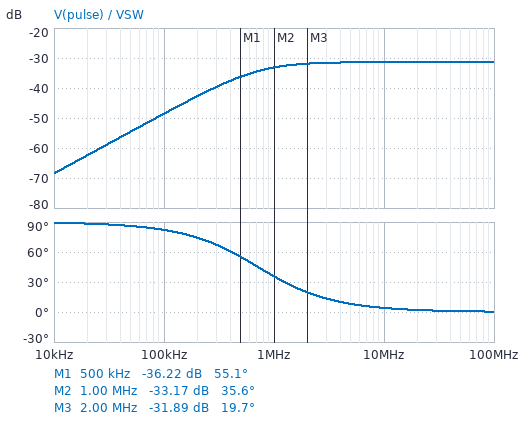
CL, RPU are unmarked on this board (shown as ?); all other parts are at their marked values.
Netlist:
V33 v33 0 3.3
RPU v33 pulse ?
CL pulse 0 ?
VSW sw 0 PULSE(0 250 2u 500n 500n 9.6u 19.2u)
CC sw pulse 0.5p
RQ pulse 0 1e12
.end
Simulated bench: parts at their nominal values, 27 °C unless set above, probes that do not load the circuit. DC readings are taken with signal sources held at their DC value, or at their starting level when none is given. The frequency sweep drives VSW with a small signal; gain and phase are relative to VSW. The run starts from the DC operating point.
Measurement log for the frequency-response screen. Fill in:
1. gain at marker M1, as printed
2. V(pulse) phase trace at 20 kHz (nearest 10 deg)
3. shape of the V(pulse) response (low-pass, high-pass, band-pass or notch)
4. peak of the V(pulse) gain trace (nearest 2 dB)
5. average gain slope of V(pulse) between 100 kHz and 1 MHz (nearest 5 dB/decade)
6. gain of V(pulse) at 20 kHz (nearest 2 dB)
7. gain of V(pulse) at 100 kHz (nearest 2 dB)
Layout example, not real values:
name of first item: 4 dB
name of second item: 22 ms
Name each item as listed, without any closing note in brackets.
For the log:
gain at marker M1, as printed: -36.22 dB
V(pulse) phase trace at 20 kHz: 90 deg
shape of the V(pulse) response: high-pass
peak of the V(pulse) gain trace: -32 dB
average gain slope of V(pulse) between 100 kHz and 1 MHz: 15 dB/decade
gain of V(pulse) at 20 kHz: -62 dB
gain of V(pulse) at 100 kHz: -48 dB
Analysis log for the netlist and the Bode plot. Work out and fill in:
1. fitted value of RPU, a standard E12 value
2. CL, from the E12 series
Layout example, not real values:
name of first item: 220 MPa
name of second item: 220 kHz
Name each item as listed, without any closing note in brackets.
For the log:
fitted value of RPU, a standard E12 value: 12 kΩ
CL, from the E12 series: 18 pF
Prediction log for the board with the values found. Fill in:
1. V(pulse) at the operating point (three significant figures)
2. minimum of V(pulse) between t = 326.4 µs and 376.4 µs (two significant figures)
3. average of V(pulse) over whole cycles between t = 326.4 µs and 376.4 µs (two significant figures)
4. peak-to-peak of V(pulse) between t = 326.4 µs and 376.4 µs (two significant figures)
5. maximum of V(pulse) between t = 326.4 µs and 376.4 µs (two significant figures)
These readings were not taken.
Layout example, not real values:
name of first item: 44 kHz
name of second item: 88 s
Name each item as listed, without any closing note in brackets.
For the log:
V(pulse) at the operating point: 3.30 V
minimum of V(pulse) between t = 326.4 µs and 376.4 µs: 610 mV
average of V(pulse) over whole cycles between t = 326.4 µs and 376.4 µs: 3.3 V
peak-to-peak of V(pulse) between t = 326.4 µs and 376.4 µs: 5.4 V
maximum of V(pulse) between t = 326.4 µs and 376.4 µs: 6.0 V
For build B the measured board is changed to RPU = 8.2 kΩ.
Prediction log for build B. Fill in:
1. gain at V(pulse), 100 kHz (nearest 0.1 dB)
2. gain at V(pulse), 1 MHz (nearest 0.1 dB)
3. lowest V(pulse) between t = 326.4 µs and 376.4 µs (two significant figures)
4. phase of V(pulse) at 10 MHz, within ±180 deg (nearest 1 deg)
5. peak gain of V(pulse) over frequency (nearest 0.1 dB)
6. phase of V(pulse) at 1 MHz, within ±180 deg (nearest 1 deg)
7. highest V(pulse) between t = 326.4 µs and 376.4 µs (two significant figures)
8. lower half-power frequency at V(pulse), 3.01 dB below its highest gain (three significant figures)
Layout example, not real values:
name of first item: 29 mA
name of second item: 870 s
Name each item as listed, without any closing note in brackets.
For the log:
gain at V(pulse), 100 kHz: -51.8 dB
gain at V(pulse), 1 MHz: -34.6 dB
lowest V(pulse) between t = 326.4 µs and 376.4 µs: 1.3 V
phase of V(pulse) at 10 MHz, within ±180 deg: 6 deg
peak gain of V(pulse) over frequency: -31.4 dB
phase of V(pulse) at 1 MHz, within ±180 deg: 46 deg
highest V(pulse) between t = 326.4 µs and 376.4 µs: 5.3 V
lower half-power frequency at V(pulse), 3.01 dB below its highest gain: 1.05 MHz
